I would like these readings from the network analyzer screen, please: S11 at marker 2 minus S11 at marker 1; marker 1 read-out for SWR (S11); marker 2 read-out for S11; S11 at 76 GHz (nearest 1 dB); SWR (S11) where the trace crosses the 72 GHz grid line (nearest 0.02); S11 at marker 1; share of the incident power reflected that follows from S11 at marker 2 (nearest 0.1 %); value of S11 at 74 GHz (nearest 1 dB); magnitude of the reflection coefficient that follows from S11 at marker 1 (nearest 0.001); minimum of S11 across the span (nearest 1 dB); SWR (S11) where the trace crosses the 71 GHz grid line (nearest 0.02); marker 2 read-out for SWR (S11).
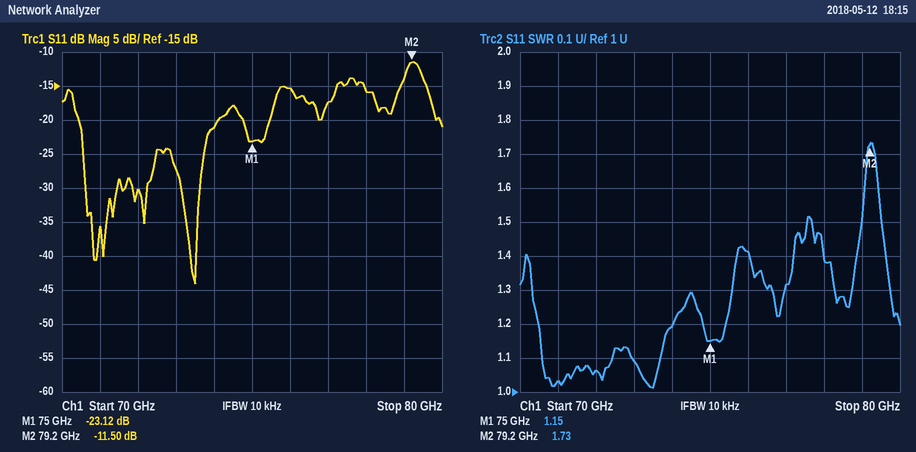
11.62 dB
1.15
-11.50 dB
-15 dB
1.06
-23.12 dB
7.1 %
-21 dB
0.070
-44 dB
1.04
1.73
